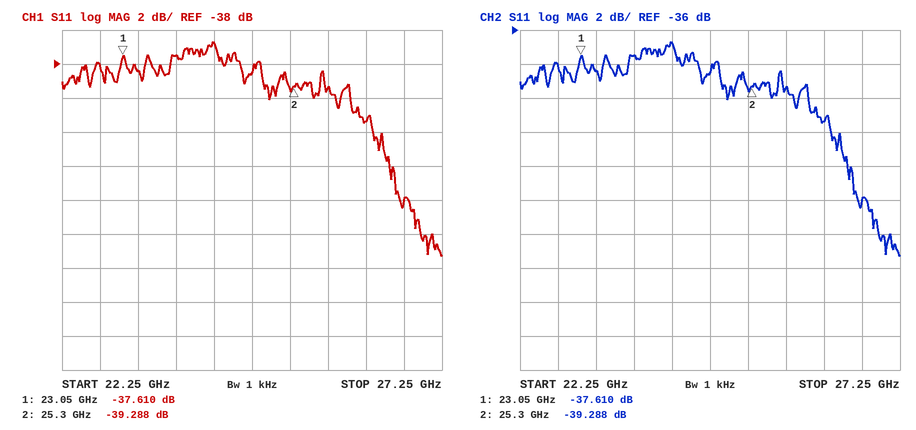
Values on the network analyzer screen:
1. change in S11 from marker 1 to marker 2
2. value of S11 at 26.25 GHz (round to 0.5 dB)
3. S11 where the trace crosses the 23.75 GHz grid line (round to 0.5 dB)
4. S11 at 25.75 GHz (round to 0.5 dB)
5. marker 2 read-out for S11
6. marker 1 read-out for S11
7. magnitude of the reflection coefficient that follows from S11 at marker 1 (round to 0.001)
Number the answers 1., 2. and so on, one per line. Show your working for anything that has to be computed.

1. -39.288 − (-37.61) = -1.678 dB
2. -41.5 dB
3. -37.5 dB
4. -39.5 dB
5. -39.288 dB
6. -37.610 dB
7. 10^(-37.61/20) ≈ 0.013
